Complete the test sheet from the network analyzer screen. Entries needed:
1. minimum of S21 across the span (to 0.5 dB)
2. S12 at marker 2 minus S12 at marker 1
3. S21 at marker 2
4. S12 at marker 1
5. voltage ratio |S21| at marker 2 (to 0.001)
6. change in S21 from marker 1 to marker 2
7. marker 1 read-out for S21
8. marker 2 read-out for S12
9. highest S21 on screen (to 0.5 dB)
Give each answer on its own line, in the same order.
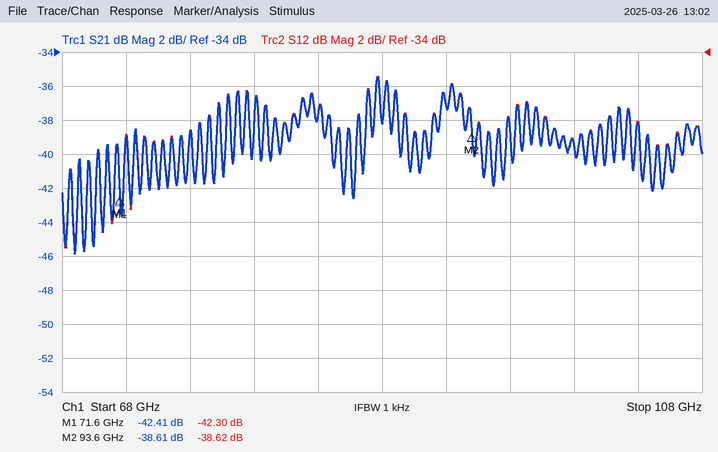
-46.0 dB
3.68 dB
-38.61 dB
-42.30 dB
0.012
3.80 dB
-42.41 dB
-38.62 dB
-35.5 dB
